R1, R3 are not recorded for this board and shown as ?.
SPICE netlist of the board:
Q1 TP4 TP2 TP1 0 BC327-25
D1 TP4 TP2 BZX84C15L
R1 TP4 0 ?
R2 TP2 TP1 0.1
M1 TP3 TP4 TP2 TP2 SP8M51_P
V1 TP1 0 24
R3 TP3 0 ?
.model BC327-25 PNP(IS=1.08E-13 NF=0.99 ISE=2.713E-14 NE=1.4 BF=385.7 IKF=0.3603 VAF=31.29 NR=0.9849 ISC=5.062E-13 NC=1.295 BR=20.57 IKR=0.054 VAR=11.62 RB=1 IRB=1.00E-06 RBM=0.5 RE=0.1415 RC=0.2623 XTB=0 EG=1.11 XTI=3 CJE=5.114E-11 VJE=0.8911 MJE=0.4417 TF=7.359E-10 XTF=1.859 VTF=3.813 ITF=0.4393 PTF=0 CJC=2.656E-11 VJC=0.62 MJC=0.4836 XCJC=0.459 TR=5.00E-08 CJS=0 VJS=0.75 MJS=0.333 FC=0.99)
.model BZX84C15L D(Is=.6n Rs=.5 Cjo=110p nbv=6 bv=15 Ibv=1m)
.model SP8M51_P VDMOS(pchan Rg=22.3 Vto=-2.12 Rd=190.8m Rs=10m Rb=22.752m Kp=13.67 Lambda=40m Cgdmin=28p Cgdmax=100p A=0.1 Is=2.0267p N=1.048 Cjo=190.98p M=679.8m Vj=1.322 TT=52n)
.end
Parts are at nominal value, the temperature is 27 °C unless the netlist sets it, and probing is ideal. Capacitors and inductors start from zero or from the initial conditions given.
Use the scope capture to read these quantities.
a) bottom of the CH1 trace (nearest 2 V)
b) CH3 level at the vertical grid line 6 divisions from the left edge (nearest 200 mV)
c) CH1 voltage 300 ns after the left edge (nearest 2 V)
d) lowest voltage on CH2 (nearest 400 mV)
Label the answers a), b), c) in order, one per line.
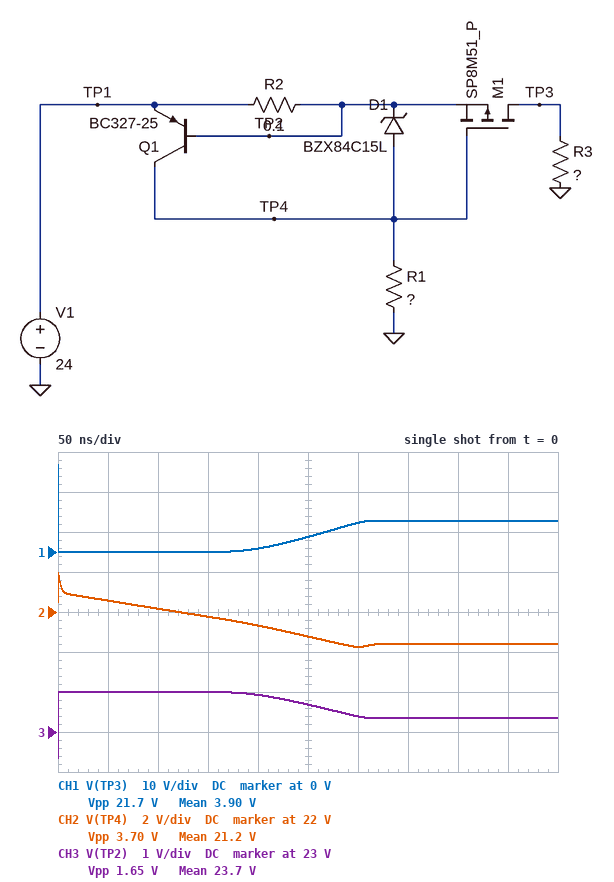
a) 0 V
b) 23.4 V
c) 8 V
d) 20.4 V
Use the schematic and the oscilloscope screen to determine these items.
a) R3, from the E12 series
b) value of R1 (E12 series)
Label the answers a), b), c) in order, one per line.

a) 1.2 Ω
b) 1.8 kΩ
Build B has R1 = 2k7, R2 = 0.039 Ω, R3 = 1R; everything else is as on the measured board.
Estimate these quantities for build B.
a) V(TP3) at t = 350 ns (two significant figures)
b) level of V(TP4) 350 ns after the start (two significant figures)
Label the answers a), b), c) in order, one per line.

a) 2.5 V
b) 21 V
